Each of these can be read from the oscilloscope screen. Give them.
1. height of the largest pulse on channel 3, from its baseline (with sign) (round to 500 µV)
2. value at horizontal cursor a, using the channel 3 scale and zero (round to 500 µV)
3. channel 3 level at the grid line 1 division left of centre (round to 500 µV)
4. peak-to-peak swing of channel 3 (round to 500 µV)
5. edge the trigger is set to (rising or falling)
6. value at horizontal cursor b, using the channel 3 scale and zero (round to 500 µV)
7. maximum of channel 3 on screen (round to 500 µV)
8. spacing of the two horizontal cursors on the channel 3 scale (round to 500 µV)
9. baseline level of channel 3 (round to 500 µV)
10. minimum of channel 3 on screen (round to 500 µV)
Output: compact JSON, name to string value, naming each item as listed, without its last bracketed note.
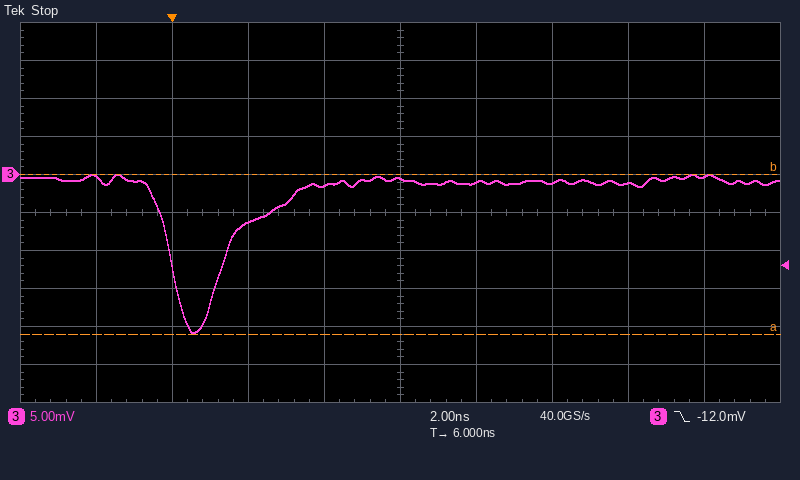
{"height of the largest pulse on channel 3, from its baseline (with sign)": "-20.0 mV", "value at horizontal cursor a, using the channel 3 scale and zero": "-21.0 mV", "channel 3 level at the grid line 1 division left of centre": "-1.5 mV", "peak-to-peak swing of channel 3": "21.0 mV", "edge the trigger is set to": "falling", "value at horizontal cursor b, using the channel 3 scale and zero": "0.0 mV", "maximum of channel 3 on screen": "0.0 mV", "spacing of the two horizontal cursors on the channel 3 scale": "21.0 mV", "baseline level of channel 3": "-1.0 mV", "minimum of channel 3 on screen": "-21.0 mV"}
